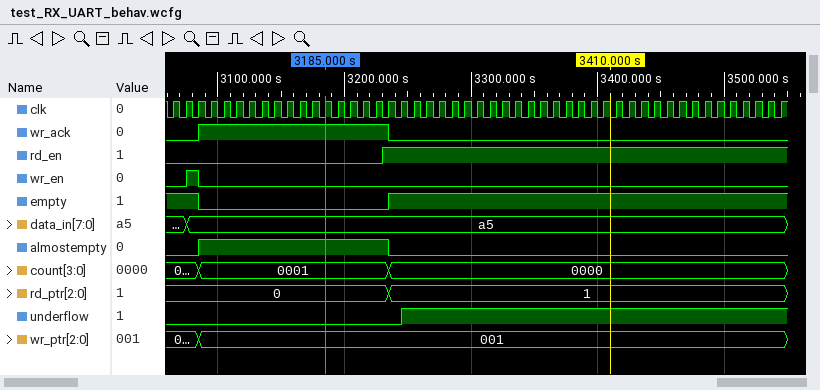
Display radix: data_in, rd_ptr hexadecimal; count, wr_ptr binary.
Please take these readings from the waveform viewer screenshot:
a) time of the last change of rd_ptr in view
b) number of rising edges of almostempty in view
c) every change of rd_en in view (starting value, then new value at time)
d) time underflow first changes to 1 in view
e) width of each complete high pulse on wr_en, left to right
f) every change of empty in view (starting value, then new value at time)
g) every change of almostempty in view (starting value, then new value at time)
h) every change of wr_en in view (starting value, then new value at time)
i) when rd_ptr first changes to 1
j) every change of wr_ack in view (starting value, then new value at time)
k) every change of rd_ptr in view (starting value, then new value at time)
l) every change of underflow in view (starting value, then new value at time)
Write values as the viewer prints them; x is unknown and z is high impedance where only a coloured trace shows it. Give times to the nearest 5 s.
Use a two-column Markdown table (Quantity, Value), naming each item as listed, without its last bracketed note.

| Quantity | Value |
|---|---|
| time of the last change of rd_ptr in view | 3235 s |
| number of rising edges of almostempty in view | 1 |
| every change of rd_en in view | 0, 1 at 3230 s |
| time underflow first changes to 1 in view | 3245 s |
| width of each complete high pulse on wr_en, left to right | 10 s |
| every change of empty in view | 1, 0 at 3085 s, 1 at 3235 s |
| every change of almostempty in view | 0, 1 at 3085 s, 0 at 3235 s |
| every change of wr_en in view | 0, 1 at 3075 s, 0 at 3085 s |
| when rd_ptr first changes to 1 | 3235 s |
| every change of wr_ack in view | 0, 1 at 3085 s, 0 at 3235 s |
| every change of rd_ptr in view | 0, 1 at 3235 s |
| every change of underflow in view | 0, 1 at 3245 s |
